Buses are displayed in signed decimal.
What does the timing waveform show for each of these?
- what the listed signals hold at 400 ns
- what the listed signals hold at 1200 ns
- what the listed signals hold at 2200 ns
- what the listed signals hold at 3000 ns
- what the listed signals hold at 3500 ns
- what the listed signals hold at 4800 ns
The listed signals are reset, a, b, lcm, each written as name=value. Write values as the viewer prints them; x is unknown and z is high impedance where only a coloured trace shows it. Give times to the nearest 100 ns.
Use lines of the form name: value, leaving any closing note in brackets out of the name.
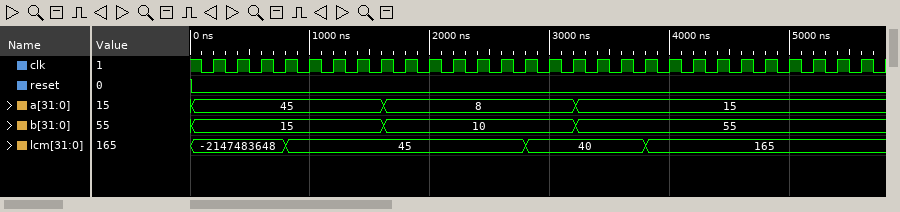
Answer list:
what the listed signals hold at 400 ns: reset=0, a=45, b=15, lcm=-2147483648
what the listed signals hold at 1200 ns: reset=0, a=45, b=15, lcm=45
what the listed signals hold at 2200 ns: reset=0, a=8, b=10, lcm=45
what the listed signals hold at 3000 ns: reset=0, a=8, b=10, lcm=40
what the listed signals hold at 3500 ns: reset=0, a=15, b=55, lcm=40
what the listed signals hold at 4800 ns: reset=0, a=15, b=55, lcm=165
